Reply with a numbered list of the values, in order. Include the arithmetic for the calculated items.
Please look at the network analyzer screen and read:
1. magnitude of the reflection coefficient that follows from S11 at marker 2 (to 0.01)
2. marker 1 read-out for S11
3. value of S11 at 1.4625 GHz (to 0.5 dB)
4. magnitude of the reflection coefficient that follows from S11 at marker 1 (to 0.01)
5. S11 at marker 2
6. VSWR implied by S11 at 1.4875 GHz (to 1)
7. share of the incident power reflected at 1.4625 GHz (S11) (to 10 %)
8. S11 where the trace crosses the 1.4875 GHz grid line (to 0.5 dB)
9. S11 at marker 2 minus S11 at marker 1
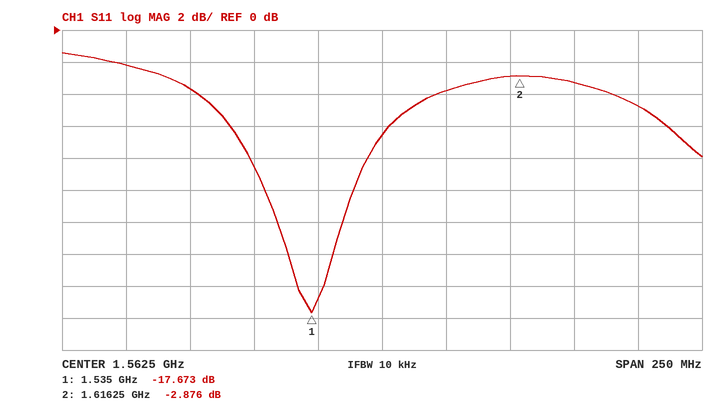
1. 10^(-2.876/20) ≈ 0.72
2. -17.673 dB
3. -2.0 dB
4. 10^(-17.673/20) ≈ 0.13
5. -2.876 dB
6. |Γ| = 10^(-3.5/20) = 0.6683; VSWR = (1 + 0.6683)/(1 − 0.6683) ≈ 5
7. 10^(-2/10) ≈ 63.1 %, so 60 % to the nearest 10 %
8. -3.5 dB
9. -2.876 − (-17.673) = 14.797 dB
